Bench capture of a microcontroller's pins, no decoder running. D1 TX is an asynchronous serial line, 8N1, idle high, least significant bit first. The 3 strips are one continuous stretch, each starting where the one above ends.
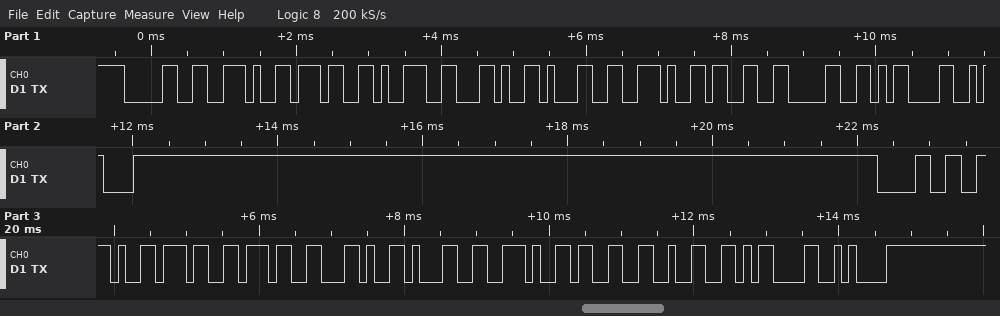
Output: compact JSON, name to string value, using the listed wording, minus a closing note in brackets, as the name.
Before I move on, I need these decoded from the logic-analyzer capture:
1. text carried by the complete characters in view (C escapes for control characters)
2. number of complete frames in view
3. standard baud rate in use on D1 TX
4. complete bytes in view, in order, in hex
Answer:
{"text carried by the complete characters in view": "\"0.79,1.30\\r\\n0.77,1.32\\r\\n\"", "number of complete frames in view": "22", "standard baud rate in use on D1 TX": "9600 baud", "complete bytes in view, in order, in hex": "30 2E 37 39 2C 31 2E 33 30 0D 0A 30 2E 37 37 2C 31 2E 33 32 0D 0A"}
